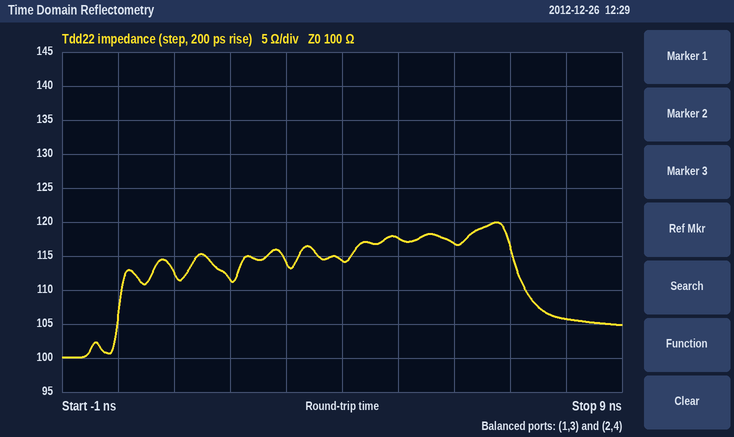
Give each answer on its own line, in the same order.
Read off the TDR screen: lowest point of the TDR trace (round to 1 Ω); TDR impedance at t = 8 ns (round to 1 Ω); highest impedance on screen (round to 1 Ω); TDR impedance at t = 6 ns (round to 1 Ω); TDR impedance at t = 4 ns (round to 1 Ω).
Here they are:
100 Ω
106 Ω
120 Ω
117 Ω
114 Ω
